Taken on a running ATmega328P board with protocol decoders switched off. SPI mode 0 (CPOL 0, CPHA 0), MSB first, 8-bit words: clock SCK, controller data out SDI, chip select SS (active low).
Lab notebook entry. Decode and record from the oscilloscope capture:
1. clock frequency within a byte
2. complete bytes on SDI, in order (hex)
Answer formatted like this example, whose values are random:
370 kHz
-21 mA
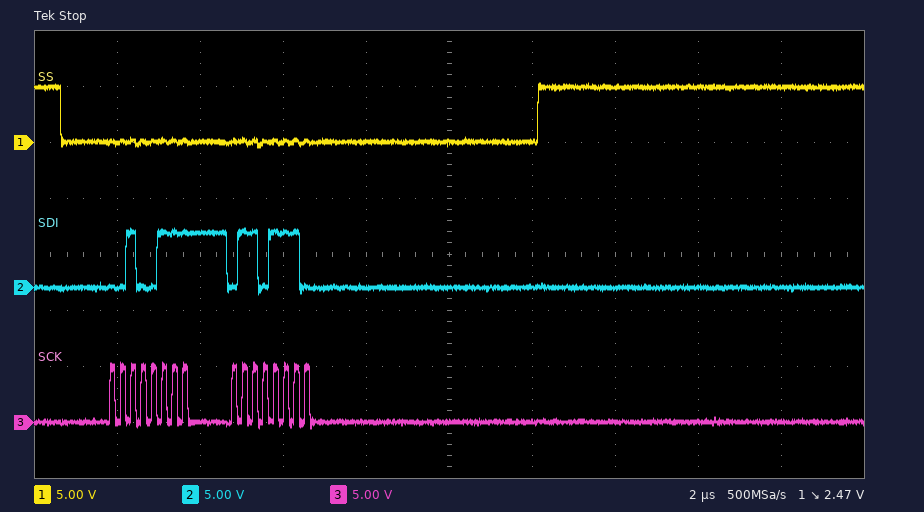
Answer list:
4 MHz
27 6E
